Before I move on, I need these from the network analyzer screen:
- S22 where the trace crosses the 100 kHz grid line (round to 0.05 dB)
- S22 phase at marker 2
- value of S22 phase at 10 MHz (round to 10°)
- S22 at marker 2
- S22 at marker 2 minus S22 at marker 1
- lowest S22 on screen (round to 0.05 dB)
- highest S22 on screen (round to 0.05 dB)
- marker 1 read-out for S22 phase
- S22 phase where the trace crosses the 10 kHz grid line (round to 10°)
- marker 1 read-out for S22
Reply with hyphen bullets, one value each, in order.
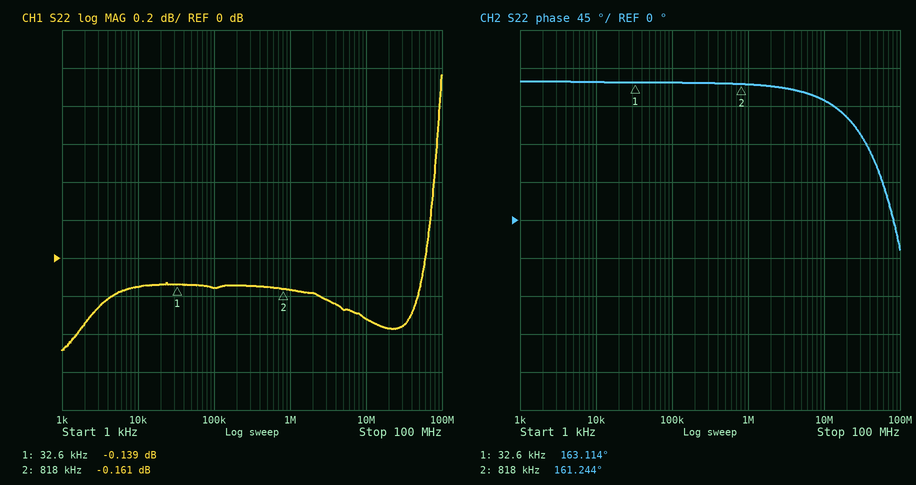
- -0.15 dB
- 161.244°
- 140°
- -0.161 dB
- -0.022 dB
- -0.50 dB
- 0.95 dB
- 163.114°
- 160°
- -0.139 dB
